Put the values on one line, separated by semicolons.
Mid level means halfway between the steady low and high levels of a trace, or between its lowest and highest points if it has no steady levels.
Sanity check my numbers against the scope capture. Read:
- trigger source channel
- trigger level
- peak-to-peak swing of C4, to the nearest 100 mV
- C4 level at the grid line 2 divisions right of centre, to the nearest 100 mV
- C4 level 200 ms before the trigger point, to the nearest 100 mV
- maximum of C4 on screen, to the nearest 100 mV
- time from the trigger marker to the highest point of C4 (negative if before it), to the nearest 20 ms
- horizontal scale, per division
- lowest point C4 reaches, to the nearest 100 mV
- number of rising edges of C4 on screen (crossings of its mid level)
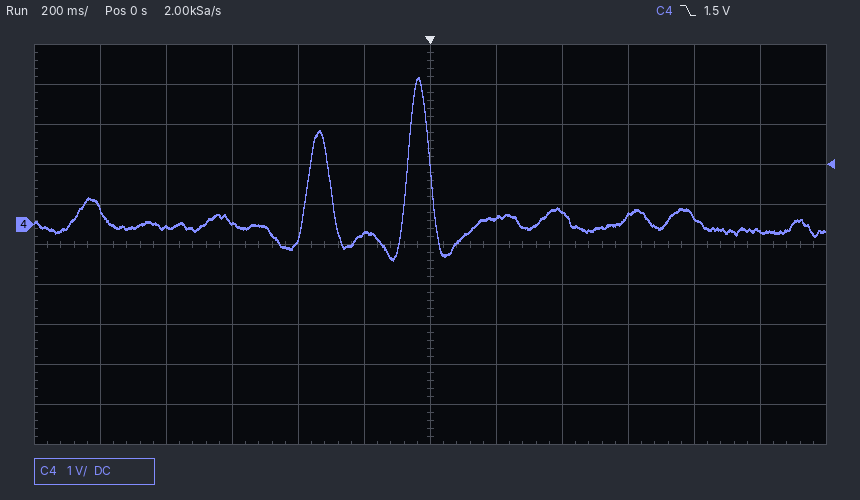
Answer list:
C4; 1.5 V; 4.6 V; 300 mV; -200 mV; 3.7 V; -40 ms; 200 ms; -900 mV; 2
